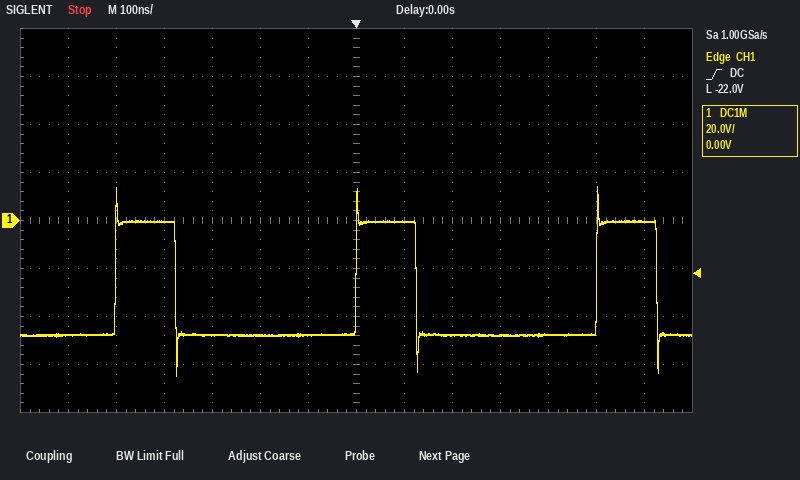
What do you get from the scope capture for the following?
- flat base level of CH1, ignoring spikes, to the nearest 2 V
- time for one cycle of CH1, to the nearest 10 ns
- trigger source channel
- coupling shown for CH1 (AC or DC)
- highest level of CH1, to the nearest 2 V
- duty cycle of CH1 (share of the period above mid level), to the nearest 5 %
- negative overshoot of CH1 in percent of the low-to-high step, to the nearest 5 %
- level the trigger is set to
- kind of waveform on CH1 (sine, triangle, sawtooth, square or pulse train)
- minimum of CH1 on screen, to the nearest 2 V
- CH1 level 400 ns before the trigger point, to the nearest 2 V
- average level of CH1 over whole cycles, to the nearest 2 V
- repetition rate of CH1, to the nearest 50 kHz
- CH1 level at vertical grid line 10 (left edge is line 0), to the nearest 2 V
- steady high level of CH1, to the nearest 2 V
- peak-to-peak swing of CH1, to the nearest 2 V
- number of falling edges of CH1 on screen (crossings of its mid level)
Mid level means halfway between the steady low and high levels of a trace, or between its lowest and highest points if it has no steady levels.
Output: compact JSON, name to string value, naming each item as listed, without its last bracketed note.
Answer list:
{"flat base level of CH1, ignoring spikes, to the nearest 2 V": "-48 V", "time for one cycle of CH1, to the nearest 10 ns": "500 ns", "trigger source channel": "CH1", "coupling shown for CH1": "DC", "highest level of CH1, to the nearest 2 V": "14 V", "duty cycle of CH1 (share of the period above mid level), to the nearest 5 %": "25 %", "negative overshoot of CH1 in percent of the low-to-high step, to the nearest 5 %": "35 %", "level the trigger is set to": "-22.0 V", "kind of waveform on CH1": "pulse train", "minimum of CH1 on screen, to the nearest 2 V": "-64 V", "CH1 level 400 ns before the trigger point, to the nearest 2 V": "0 V", "average level of CH1 over whole cycles, to the nearest 2 V": "-36 V", "repetition rate of CH1, to the nearest 50 kHz": "2.00 MHz", "CH1 level at vertical grid line 10 (left edge is line 0), to the nearest 2 V": "-48 V", "steady high level of CH1, to the nearest 2 V": "0 V", "peak-to-peak swing of CH1, to the nearest 2 V": "78 V", "number of falling edges of CH1 on screen": "3"}
